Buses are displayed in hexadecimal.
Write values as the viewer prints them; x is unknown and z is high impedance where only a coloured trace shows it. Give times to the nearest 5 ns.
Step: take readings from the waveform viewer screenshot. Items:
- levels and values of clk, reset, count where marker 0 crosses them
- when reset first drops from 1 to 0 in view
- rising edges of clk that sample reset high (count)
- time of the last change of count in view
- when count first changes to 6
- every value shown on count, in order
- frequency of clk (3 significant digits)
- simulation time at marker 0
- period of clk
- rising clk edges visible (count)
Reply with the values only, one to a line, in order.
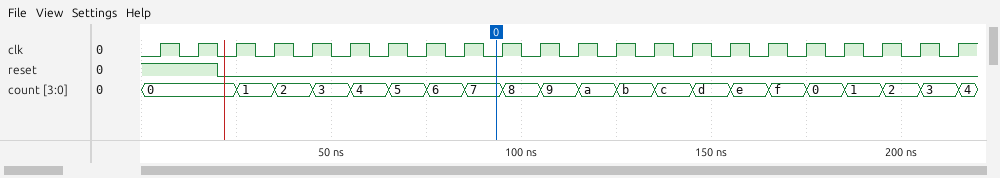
clk=0, reset=0, count=7
20 ns
2
215 ns
75 ns
0, 1, 2, 3, 4, 5, 6, 7, 8, 9, a, b, c, d, e, f, 0, 1, 2, 3, 4
100 MHz
95 ns
10 ns
22
